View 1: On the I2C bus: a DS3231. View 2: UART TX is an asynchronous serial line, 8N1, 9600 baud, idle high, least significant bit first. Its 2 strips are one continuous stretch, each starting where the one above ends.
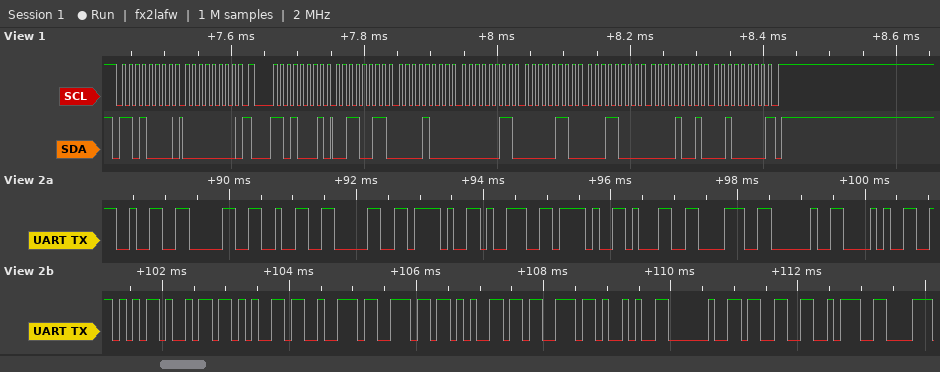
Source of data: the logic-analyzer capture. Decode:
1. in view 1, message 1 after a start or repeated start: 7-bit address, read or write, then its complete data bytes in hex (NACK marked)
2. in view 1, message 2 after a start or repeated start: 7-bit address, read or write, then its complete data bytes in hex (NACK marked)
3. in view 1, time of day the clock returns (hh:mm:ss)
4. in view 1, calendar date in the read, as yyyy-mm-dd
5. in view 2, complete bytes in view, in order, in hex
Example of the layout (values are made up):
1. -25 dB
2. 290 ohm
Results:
1. 0x68 write: 00
2. 0x68 read: 33 08 03 06 18 09 20 NACK
3. 03:08:33
4. 2020-09-18
5. 0x32 0x30 0x32 0x30 0x2F 0x39 0x2F 0x31 0x38 0x20 0x28 0x56 0x69 0x65 0x72 0x6E 0x65 0x73 0x29 0x20 0x33 0x3A
